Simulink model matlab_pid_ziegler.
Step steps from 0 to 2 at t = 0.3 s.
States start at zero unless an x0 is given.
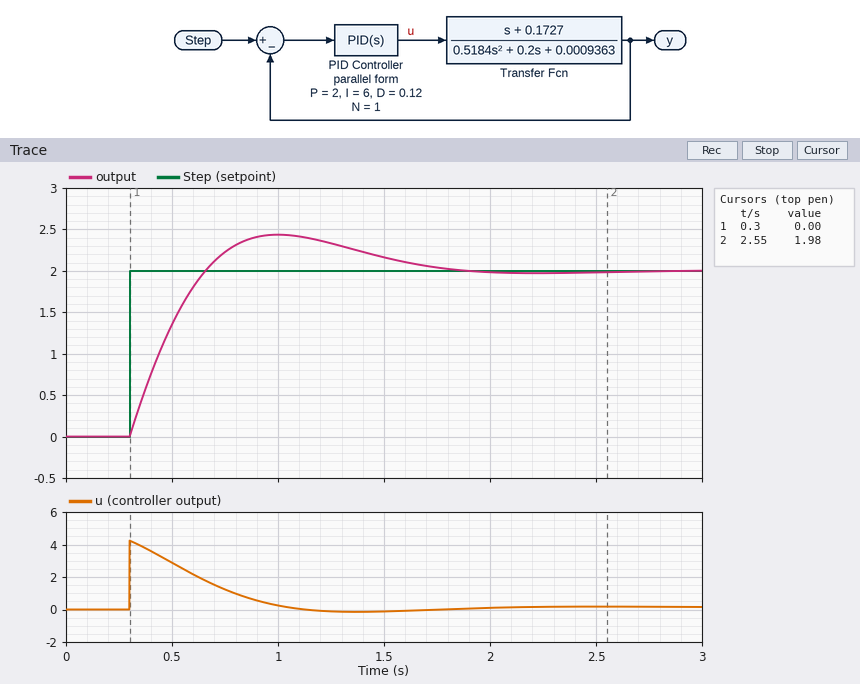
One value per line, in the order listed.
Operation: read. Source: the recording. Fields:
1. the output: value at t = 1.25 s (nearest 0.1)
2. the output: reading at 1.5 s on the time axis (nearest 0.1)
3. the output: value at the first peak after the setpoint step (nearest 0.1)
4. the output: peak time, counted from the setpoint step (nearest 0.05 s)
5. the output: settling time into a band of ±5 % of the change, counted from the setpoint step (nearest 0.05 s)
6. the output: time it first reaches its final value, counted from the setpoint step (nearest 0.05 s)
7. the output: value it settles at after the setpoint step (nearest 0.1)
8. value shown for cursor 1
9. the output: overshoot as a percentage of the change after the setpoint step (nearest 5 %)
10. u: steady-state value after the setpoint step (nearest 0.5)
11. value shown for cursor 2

2.3
2.2
2.4
0.70 s
1.30 s
0.35 s
2.0
0.00
20 %
0.0
1.98
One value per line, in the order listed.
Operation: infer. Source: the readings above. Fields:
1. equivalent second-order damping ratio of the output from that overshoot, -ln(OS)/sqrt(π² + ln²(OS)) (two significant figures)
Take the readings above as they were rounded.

0.46
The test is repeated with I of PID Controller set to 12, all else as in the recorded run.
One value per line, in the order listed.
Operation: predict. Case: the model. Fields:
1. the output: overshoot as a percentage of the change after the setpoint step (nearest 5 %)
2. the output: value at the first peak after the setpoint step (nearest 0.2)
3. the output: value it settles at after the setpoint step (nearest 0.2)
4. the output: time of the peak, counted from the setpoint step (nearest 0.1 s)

30 %
2.6
2.0
0.5 s
